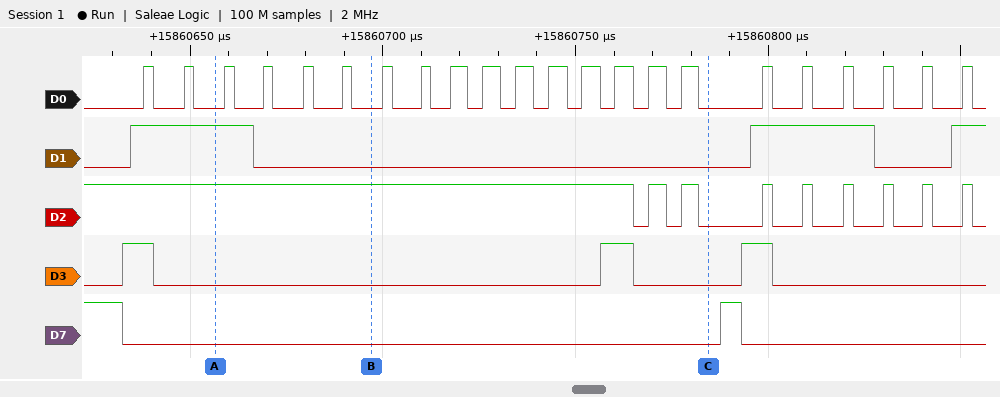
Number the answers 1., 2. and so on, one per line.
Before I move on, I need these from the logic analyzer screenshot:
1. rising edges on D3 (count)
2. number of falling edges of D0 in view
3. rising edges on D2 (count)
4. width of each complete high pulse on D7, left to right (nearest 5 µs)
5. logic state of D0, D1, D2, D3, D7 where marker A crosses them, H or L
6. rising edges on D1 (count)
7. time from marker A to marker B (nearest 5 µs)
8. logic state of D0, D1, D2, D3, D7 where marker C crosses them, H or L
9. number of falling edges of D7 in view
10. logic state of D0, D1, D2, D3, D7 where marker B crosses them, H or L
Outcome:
1. 3
2. 22
3. 8
4. 5 µs
5. D0=L, D1=H, D2=H, D3=L, D7=L
6. 3
7. 40 µs
8. D0=L, D1=L, D2=L, D3=L, D7=L
9. 2
10. D0=L, D1=L, D2=H, D3=L, D7=L
